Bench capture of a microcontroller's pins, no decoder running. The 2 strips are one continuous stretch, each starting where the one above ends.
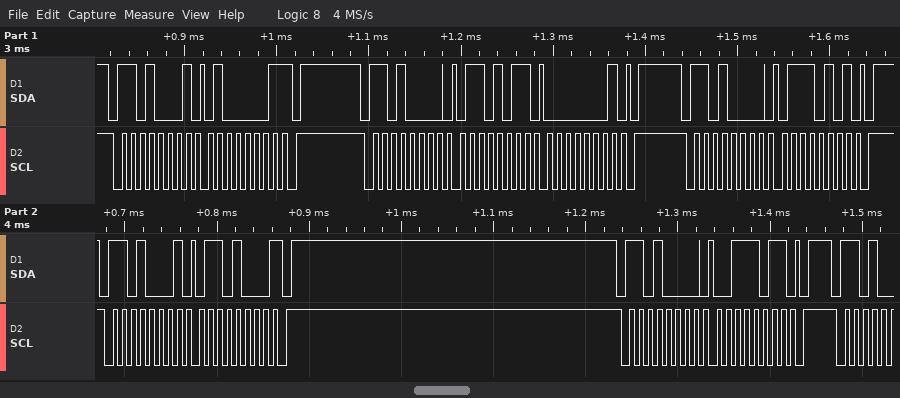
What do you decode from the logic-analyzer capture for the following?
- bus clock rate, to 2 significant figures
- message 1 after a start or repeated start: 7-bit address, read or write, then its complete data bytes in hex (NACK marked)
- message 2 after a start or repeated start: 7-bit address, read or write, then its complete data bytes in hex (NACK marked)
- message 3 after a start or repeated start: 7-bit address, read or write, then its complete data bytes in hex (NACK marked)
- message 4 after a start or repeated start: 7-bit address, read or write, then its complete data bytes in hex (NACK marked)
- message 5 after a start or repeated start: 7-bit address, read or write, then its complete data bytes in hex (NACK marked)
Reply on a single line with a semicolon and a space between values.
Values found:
100 kHz; 0x68 read: 41 NACK; 0x68 write: 6B 01; 0x68 write: 75; 0x68 read: 68 NACK; 0x68 write: 3B
